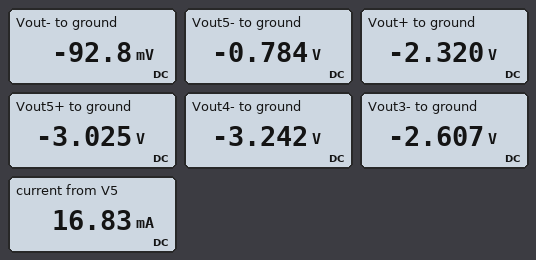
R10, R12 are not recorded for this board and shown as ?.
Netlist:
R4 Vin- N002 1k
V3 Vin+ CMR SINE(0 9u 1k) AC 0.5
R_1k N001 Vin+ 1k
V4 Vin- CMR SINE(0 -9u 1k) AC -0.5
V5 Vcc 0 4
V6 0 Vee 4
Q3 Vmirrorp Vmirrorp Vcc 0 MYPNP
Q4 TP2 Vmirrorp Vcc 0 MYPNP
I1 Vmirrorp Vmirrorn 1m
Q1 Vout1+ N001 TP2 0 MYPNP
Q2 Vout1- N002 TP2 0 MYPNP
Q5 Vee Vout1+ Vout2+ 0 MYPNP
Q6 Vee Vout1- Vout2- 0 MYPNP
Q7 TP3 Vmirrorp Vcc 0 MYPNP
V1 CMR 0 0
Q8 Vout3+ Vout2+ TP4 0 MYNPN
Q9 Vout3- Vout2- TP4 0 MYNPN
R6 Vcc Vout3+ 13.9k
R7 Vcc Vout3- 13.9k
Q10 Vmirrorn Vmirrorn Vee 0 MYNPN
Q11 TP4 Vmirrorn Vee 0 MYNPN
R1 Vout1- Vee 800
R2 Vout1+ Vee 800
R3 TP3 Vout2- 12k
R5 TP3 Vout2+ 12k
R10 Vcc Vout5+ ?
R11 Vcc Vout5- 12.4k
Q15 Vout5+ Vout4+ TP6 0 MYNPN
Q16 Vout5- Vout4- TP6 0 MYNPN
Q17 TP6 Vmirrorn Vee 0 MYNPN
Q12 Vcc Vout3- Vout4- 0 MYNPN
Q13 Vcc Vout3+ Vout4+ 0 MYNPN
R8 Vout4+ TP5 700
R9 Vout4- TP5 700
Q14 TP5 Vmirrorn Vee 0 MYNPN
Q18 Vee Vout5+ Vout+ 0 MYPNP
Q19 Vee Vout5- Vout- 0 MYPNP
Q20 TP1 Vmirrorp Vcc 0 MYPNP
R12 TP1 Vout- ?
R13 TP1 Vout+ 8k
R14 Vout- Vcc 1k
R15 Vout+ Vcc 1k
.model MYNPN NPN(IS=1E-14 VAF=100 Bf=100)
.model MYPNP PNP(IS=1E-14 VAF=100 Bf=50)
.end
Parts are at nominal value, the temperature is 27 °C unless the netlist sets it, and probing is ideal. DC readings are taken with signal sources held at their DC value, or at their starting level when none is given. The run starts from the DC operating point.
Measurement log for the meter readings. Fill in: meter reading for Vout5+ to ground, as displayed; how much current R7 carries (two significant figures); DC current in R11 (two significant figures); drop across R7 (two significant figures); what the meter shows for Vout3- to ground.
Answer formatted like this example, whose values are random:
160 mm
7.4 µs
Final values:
-3.025 V
480 µA
390 µA
6.6 V
-2.607 V
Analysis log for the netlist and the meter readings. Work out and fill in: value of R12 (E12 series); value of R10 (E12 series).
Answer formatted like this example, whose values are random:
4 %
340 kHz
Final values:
22 kΩ
22 kΩ
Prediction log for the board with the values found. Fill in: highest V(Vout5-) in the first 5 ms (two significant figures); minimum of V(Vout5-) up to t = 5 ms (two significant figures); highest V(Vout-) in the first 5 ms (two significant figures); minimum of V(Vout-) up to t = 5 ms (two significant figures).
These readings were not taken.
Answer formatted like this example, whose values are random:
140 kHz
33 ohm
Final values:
750 mV
-3.2 V
1.4 V
-2.5 V
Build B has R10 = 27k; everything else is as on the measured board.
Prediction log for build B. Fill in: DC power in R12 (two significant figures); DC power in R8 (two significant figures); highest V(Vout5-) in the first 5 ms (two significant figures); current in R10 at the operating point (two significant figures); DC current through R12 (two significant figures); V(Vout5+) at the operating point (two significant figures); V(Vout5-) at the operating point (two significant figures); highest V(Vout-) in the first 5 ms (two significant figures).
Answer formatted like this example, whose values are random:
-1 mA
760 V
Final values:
510 µW
160 µW
370 mV
290 µA
150 µA
-3.8 V
-890 mV
1.1 V
